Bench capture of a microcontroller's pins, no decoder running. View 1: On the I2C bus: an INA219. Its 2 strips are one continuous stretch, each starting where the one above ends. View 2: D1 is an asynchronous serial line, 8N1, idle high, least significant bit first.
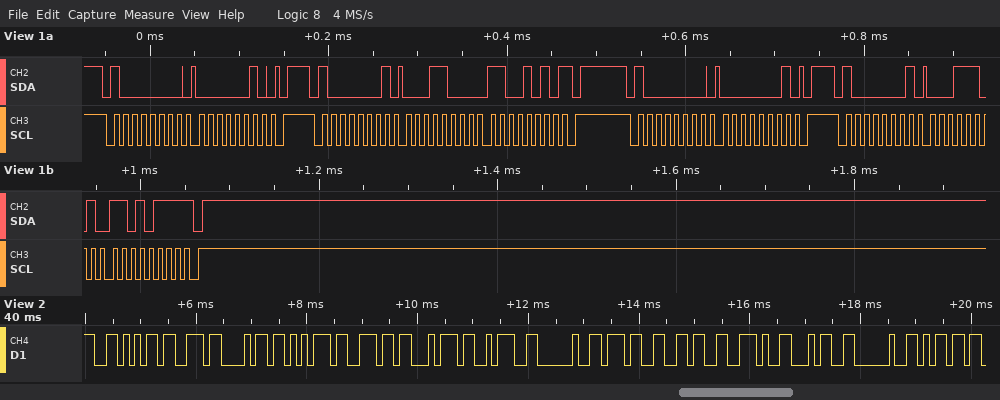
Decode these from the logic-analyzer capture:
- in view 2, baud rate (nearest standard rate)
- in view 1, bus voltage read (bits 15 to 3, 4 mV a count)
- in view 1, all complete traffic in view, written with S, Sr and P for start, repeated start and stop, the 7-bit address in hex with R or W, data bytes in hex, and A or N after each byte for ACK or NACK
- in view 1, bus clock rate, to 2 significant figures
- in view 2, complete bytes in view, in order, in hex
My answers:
9600 baud
3.172 V
S 40W A 02 A P S 40R A 18 A CA N P S 40W A 01 A P S 40R A 1D A D7 N P
100 kHz
0x56 0x73 0x68 0x75 0x6E 0x74 0x3A 0x20 0x37 0x36 0x2E 0x34 0x20 0x6D
